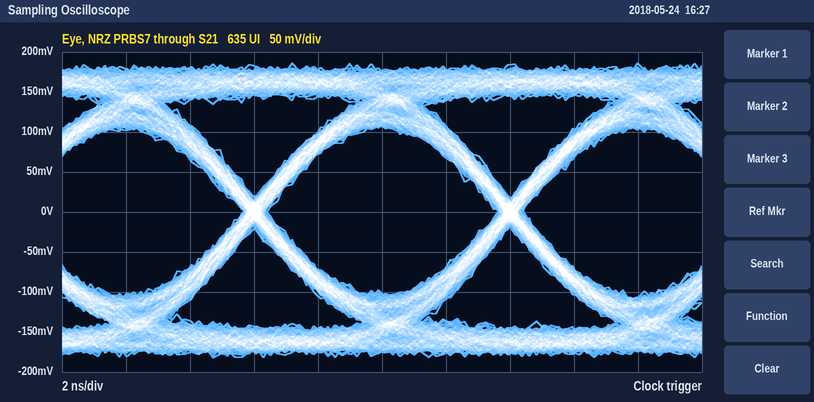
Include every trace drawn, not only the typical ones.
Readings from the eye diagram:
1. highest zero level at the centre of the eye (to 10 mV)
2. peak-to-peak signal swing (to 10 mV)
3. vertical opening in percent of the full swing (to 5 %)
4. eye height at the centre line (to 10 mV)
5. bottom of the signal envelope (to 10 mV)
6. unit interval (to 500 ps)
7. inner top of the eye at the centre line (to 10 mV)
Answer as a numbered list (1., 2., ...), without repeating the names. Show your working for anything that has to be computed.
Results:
1. -100 mV
2. 370 mV
3. 210 mV / 370 mV ≈ 56.8 %, so 55 % to the nearest 5 %
4. 210 mV
5. -180 mV
6. 8.0 ns
7. 110 mV
